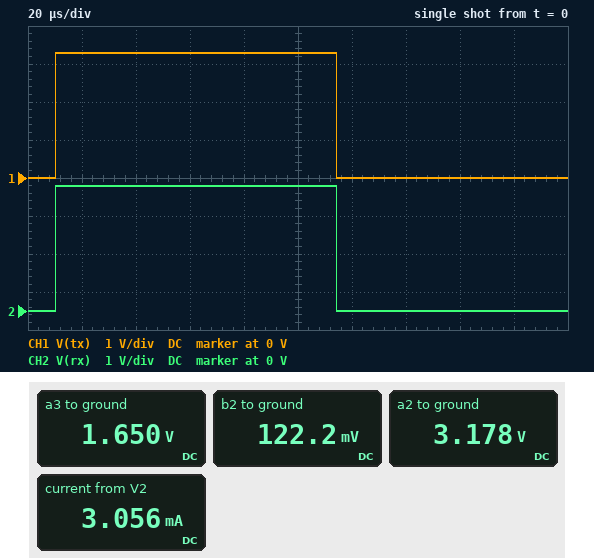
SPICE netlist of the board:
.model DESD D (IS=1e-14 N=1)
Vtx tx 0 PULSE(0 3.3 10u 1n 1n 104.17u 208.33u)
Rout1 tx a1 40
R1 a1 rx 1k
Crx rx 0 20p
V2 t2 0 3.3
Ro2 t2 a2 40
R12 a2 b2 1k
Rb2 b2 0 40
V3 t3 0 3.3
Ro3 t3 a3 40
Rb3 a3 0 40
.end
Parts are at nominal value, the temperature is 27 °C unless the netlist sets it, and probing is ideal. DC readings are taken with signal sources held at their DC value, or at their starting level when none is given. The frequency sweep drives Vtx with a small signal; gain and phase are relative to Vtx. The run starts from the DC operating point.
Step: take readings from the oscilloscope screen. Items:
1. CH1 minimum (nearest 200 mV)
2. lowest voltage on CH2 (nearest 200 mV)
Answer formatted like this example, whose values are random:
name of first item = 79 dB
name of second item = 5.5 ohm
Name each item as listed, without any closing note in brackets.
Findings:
CH1 minimum = 0 V
lowest voltage on CH2 = 0 V
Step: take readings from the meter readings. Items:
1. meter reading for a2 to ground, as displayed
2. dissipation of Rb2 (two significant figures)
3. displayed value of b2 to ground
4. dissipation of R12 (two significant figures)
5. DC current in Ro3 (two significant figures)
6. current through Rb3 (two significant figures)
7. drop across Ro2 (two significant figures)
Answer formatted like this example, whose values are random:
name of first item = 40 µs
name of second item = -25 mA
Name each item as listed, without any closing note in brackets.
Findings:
meter reading for a2 to ground, as displayed = 3.178 V
dissipation of Rb2 = 370 µW
displayed value of b2 to ground = 122.2 mV
dissipation of R12 = 9.3 mW
DC current in Ro3 = 41 mA
current through Rb3 = 41 mA
drop across Ro2 = 120 mV
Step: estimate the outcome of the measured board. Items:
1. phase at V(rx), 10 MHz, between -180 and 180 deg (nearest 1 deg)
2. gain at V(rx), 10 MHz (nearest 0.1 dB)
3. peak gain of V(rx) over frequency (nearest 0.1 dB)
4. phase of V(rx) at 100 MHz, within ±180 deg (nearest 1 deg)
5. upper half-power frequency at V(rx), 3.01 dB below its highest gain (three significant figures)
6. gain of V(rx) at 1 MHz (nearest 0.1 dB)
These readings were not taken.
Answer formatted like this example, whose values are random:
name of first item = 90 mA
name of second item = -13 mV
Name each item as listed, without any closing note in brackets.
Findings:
phase at V(rx), 10 MHz, between -180 and 180 deg = -53 deg
gain at V(rx), 10 MHz = -4.3 dB
peak gain of V(rx) over frequency = 0 dB
phase of V(rx) at 100 MHz, within ±180 deg = -86 deg
upper half-power frequency at V(rx), 3.01 dB below its highest gain = 7.65 MHz
gain of V(rx) at 1 MHz = -0.1 dB
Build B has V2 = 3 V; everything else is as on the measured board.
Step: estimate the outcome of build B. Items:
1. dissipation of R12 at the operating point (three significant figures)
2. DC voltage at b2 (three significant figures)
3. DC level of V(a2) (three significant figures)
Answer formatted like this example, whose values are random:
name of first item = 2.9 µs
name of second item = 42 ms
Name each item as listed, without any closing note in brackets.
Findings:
dissipation of R12 at the operating point = 7.72 mW
DC voltage at b2 = 111 mV
DC level of V(a2) = 2.89 V
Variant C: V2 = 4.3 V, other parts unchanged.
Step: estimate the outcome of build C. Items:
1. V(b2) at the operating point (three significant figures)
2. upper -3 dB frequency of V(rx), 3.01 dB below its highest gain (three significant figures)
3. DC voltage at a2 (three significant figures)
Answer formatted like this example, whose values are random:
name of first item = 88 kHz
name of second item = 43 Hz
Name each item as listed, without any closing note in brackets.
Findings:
V(b2) at the operating point = 159 mV
upper -3 dB frequency of V(rx), 3.01 dB below its highest gain = 7.65 MHz
DC voltage at a2 = 4.14 V
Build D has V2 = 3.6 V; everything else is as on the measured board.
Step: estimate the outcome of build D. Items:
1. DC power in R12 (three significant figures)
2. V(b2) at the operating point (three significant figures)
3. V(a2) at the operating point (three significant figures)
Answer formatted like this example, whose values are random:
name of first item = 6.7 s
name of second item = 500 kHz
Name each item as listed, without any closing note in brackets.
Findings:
DC power in R12 = 11.1 mW
V(b2) at the operating point = 133 mV
V(a2) at the operating point = 3.47 V
